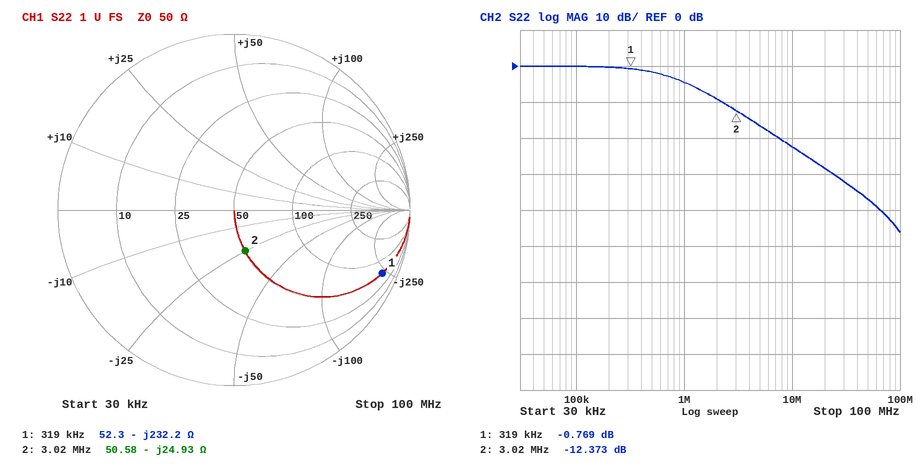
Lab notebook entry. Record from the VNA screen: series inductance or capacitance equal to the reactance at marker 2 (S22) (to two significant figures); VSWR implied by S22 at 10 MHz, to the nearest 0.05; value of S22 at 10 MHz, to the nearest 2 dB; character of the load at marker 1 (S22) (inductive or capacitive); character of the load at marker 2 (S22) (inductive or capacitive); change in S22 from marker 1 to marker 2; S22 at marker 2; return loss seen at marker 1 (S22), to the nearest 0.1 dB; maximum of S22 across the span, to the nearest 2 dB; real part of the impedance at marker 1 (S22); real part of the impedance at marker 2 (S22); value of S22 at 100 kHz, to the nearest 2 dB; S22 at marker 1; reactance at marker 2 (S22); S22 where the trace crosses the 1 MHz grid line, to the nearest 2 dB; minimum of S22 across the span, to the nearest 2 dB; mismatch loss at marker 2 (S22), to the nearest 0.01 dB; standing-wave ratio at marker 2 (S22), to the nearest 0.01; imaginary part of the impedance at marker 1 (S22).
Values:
2.1 nF
1.15
-22 dB
capacitive
capacitive
-11.604 dB
-12.373 dB
0.8 dB
0 dB
52.3 Ω
50.58 Ω
0 dB
-0.769 dB
-24.93 Ω
-4 dB
-46 dB
0.26 dB
1.63
-232.2 Ω
